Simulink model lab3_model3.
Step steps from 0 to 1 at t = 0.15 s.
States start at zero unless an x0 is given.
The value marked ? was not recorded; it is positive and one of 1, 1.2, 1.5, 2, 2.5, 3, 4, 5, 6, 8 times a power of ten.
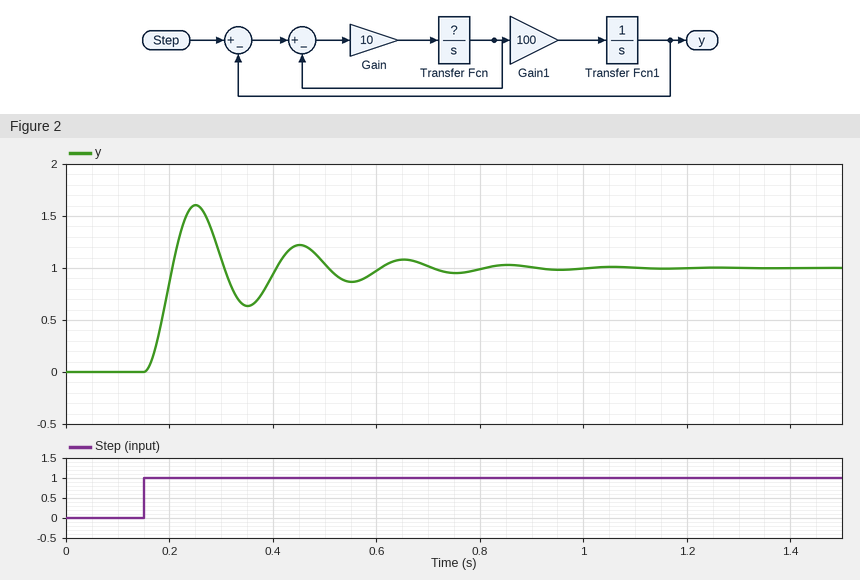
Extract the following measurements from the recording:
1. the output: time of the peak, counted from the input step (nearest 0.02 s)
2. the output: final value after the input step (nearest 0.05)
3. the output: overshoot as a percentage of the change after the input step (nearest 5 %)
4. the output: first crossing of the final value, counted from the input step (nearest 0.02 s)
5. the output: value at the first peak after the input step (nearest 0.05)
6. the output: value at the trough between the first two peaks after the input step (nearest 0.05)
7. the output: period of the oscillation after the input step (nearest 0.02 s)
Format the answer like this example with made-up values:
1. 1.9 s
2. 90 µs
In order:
1. 0.10 s
2. 1.00
3. 60 %
4. 0.06 s
5. 1.60
6. 0.65
7. 0.20 s
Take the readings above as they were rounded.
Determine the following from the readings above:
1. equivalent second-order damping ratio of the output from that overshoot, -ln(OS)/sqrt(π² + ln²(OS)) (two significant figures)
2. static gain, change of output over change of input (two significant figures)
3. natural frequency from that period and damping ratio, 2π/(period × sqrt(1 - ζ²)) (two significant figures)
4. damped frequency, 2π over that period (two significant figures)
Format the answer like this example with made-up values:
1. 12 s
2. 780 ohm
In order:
1. 0.16
2. 1.0
3. 32 rad/s
4. 31 rad/s
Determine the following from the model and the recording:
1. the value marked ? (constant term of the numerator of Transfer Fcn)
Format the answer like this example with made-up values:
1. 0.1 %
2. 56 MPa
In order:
1. 1
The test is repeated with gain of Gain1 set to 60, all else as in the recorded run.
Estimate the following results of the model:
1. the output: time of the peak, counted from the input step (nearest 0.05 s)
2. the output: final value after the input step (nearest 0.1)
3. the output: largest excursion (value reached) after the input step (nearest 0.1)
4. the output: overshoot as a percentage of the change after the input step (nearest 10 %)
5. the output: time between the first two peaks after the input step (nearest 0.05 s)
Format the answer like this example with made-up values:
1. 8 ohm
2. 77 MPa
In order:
1. 0.15 s
2. 1.0
3. 1.5
4. 50 %
5. 0.25 s
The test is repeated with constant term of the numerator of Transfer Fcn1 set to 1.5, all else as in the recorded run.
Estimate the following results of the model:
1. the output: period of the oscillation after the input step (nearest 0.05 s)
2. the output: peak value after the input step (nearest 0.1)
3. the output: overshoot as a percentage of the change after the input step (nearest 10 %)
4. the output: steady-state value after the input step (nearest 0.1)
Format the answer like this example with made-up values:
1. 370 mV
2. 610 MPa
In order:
1. 0.15 s
2. 1.7
3. 70 %
4. 1.0
